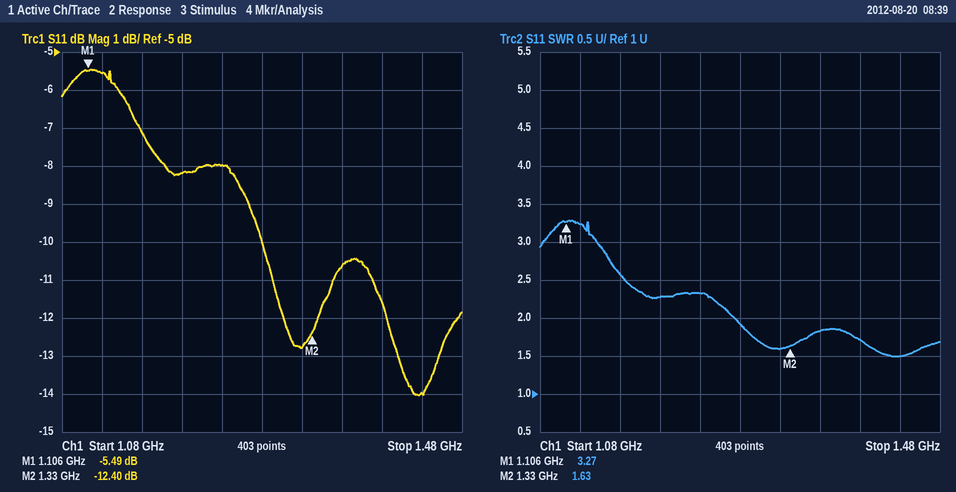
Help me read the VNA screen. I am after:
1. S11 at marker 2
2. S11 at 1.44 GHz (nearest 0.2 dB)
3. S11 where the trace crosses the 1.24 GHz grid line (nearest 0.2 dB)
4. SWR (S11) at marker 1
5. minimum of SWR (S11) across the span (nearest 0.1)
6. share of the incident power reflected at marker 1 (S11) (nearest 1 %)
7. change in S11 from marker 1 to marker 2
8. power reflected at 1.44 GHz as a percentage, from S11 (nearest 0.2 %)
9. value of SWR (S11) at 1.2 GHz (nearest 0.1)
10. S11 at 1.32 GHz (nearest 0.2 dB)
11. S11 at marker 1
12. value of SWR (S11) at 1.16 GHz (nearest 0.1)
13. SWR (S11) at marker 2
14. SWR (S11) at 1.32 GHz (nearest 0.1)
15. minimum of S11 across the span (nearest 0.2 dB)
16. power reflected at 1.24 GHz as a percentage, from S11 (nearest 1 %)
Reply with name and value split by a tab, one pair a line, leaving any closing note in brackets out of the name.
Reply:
S11 at marker 2	-12.40 dB
S11 at 1.44 GHz	-14.0 dB
S11 where the trace crosses the 1.24 GHz grid line	-8.0 dB
SWR (S11) at marker 1	3.27
minimum of SWR (S11) across the span	1.5
share of the incident power reflected at marker 1 (S11)	28 %
change in S11 from marker 1 to marker 2	-6.91 dB
power reflected at 1.44 GHz as a percentage, from S11	4.0 %
value of SWR (S11) at 1.2 GHz	2.3
S11 at 1.32 GHz	-12.8 dB
S11 at marker 1	-5.49 dB
value of SWR (S11) at 1.16 GHz	2.6
SWR (S11) at marker 2	1.63
SWR (S11) at 1.32 GHz	1.6
minimum of S11 across the span	-14.0 dB
power reflected at 1.24 GHz as a percentage, from S11	16 %
